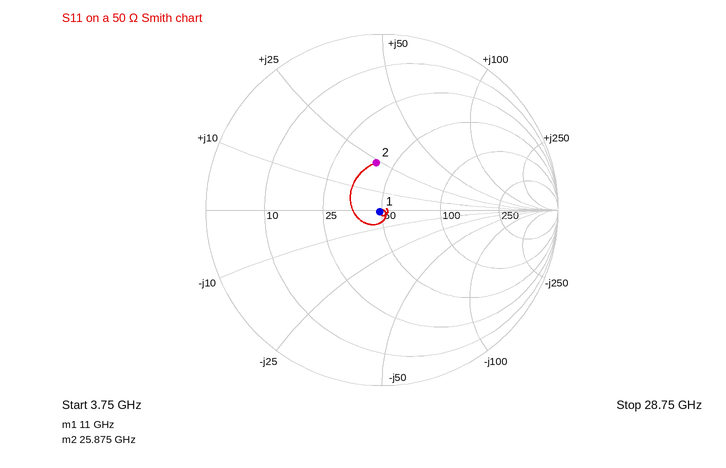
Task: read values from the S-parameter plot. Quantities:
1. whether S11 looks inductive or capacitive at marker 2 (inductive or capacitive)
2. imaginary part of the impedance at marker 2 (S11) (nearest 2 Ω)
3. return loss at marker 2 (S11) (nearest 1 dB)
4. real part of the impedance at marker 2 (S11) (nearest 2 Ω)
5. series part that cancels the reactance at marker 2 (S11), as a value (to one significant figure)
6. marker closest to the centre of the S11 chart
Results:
inductive
+24 Ω
11 dB
40 Ω
300 fF
marker 1
